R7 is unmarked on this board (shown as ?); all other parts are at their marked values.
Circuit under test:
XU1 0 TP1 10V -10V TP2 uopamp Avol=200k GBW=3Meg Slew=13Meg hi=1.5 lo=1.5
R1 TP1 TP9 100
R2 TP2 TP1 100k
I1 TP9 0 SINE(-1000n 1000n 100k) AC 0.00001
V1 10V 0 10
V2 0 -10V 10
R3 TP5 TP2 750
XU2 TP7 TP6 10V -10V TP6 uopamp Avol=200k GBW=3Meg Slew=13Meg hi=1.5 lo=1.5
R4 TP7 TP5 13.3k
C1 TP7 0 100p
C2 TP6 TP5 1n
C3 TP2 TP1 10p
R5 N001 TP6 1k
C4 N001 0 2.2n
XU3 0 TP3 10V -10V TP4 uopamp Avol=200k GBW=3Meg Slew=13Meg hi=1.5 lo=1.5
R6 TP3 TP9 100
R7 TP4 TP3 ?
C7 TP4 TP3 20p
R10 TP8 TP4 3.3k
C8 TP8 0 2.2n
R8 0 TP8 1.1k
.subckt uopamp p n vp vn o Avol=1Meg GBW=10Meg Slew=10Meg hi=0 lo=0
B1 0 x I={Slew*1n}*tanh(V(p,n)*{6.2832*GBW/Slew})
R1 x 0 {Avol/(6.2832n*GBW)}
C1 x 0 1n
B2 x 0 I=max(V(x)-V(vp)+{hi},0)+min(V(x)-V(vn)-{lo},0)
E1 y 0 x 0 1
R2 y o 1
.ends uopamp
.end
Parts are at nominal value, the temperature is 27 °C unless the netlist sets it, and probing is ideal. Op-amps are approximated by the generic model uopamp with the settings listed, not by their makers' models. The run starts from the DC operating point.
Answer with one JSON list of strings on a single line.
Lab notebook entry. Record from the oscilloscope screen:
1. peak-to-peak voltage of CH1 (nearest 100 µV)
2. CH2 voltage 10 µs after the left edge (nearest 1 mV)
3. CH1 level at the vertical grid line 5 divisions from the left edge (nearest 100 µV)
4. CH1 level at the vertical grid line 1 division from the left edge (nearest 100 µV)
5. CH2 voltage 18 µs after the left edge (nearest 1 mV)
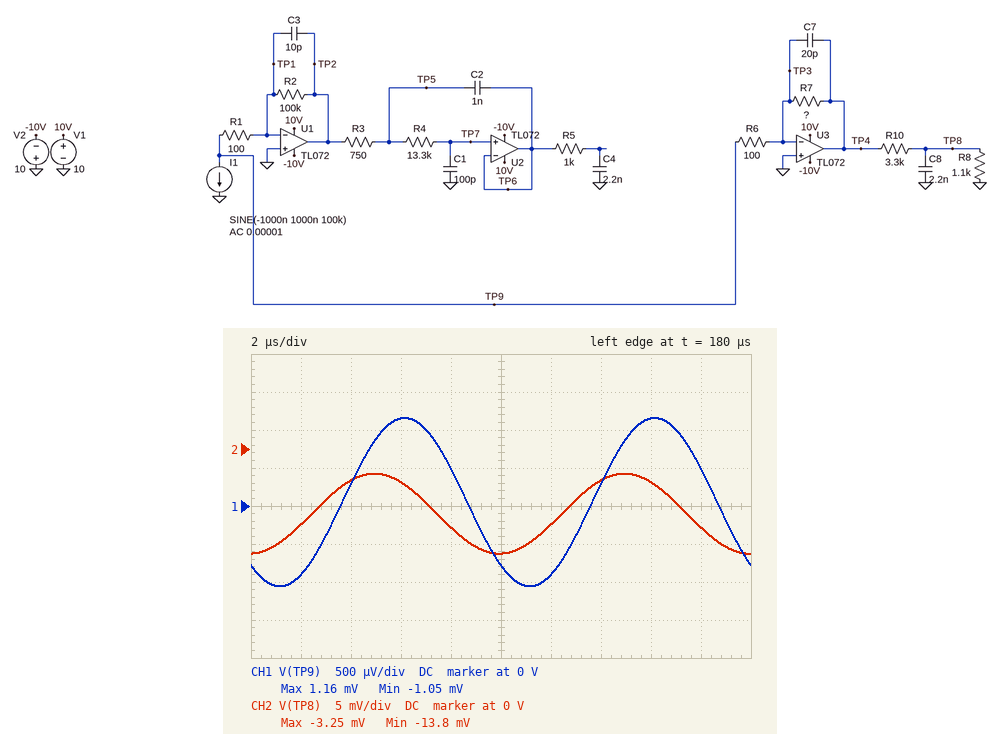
["2.2 mV", "-14 mV", "-800 µV", "-900 µV", "-10 mV"]
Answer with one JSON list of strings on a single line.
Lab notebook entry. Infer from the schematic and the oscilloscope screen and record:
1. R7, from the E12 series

["68 kΩ"]
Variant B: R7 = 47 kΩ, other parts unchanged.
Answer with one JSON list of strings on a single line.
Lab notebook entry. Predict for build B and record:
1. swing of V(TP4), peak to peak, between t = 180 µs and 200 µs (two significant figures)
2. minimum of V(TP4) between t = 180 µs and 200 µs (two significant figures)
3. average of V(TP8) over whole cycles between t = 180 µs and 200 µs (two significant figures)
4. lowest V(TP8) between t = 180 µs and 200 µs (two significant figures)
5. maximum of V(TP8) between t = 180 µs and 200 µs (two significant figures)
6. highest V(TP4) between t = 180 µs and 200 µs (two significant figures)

["54 mV", "-51 mV", "-5.9 mV", "-10 mV", "-1.4 mV", "3.6 mV"]
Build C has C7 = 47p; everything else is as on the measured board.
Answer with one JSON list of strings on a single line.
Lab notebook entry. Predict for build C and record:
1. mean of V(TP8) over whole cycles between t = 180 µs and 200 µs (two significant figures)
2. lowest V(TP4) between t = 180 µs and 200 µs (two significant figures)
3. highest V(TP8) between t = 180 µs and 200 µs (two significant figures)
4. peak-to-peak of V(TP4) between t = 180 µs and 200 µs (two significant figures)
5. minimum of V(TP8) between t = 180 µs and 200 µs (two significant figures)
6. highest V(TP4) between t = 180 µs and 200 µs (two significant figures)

["-8.5 mV", "-57 mV", "-4.8 mV", "45 mV", "-12 mV", "-11 mV"]
